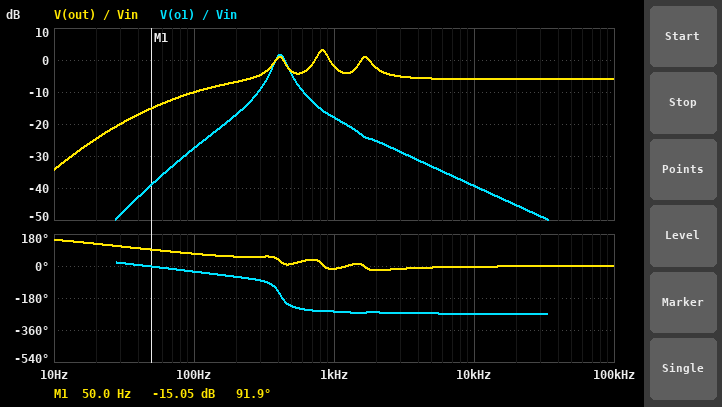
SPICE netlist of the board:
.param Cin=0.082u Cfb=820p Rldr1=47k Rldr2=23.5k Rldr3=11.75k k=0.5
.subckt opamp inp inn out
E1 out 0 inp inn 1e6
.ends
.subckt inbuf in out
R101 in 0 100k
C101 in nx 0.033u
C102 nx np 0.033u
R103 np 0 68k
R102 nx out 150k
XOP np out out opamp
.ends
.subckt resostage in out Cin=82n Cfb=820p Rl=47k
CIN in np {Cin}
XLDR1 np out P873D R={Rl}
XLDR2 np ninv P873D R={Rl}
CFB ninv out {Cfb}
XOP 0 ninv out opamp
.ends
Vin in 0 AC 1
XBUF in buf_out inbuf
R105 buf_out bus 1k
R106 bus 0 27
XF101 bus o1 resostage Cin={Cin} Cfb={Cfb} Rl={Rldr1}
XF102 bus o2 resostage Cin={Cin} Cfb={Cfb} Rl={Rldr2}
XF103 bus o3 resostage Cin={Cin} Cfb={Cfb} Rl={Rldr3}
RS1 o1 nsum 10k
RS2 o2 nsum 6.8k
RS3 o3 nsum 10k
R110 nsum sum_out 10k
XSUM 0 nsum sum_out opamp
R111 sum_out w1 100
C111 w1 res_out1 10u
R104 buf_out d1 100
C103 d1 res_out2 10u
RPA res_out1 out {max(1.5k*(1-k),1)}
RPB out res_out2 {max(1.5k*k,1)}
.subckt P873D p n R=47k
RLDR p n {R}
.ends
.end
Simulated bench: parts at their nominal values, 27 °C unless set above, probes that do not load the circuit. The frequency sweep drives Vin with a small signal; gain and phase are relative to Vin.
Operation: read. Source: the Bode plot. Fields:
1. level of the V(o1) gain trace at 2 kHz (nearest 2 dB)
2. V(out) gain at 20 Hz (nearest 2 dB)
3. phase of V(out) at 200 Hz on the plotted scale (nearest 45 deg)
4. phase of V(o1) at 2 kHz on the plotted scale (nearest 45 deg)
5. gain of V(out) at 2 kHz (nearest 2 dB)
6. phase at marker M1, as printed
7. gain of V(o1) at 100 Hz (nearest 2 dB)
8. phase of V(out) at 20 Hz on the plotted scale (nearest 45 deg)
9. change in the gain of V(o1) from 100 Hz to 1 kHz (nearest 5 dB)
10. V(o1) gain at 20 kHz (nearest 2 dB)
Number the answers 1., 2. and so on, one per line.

1. -26 dB
2. -24 dB
3. 45 deg
4. -270 deg
5. -2 dB
6. 91.9 deg
7. -28 dB
8. 135 deg
9. 10 dB
10. -46 dB
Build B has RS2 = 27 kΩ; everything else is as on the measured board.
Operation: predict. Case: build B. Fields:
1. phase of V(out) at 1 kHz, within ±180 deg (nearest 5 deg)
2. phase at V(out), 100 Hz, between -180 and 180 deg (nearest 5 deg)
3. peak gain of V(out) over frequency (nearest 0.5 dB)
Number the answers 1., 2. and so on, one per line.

1. 5 deg
2. 65 deg
3. 1.0 dB
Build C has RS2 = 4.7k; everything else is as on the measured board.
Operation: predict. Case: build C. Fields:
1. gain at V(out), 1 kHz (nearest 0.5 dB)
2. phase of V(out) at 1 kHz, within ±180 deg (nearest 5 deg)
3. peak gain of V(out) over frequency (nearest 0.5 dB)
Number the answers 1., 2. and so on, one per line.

1. -0.5 dB
2. -25 deg
3. 5.0 dB
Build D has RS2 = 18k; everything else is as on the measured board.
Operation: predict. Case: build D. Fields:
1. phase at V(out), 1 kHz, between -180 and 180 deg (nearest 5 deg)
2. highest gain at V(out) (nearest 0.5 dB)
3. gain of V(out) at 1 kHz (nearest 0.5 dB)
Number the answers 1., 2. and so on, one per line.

1. 0 deg
2. 1.0 dB
3. -4.5 dB
